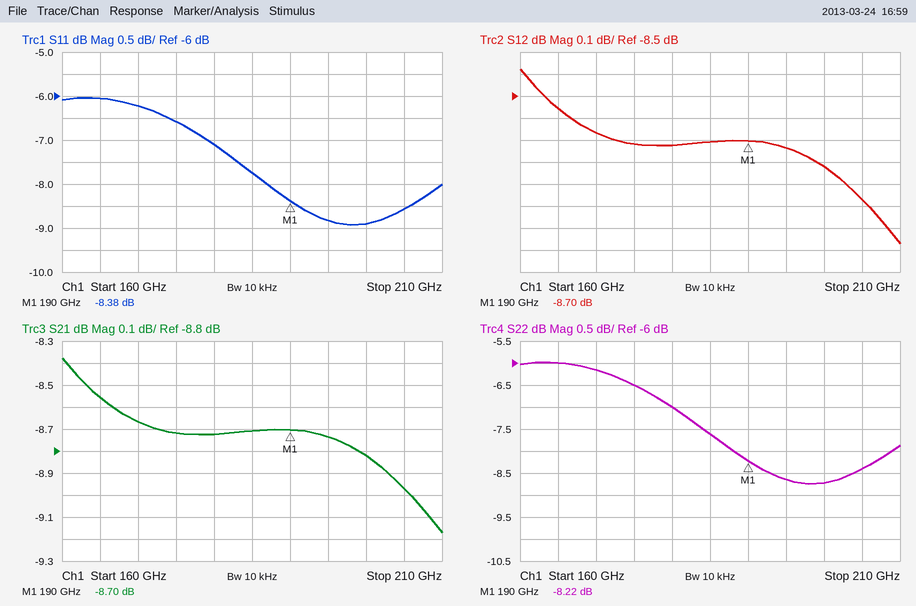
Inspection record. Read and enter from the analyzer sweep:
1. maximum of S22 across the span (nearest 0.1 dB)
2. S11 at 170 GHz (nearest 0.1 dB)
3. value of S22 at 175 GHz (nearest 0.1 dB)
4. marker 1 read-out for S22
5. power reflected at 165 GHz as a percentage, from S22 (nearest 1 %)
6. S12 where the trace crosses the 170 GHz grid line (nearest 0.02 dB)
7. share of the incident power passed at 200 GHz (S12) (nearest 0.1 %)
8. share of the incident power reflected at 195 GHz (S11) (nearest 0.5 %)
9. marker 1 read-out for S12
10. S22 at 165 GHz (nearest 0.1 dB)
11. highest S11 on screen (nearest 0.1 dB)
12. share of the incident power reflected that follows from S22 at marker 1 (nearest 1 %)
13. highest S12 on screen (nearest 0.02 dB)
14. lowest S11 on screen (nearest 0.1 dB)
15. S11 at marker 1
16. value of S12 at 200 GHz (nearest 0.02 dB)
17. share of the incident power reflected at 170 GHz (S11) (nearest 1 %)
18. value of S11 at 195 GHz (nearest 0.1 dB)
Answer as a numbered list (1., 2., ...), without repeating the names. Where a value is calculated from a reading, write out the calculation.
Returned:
1. -6.0 dB
2. -6.2 dB
3. -6.5 dB
4. -8.22 dB
5. 10^(-6/10) ≈ 25 %
6. -8.66 dB
7. 10^(-8.82/10) ≈ 13.1 %
8. 10^(-8.8/10) ≈ 13.2 %, so 13.0 % to the nearest 0.5 %
9. -8.70 dB
10. -6.0 dB
11. -6.0 dB
12. 10^(-8.22/10) ≈ 15 %
13. -8.38 dB
14. -8.9 dB
15. -8.38 dB
16. -8.82 dB
17. 10^(-6.2/10) ≈ 24 %
18. -8.8 dB
